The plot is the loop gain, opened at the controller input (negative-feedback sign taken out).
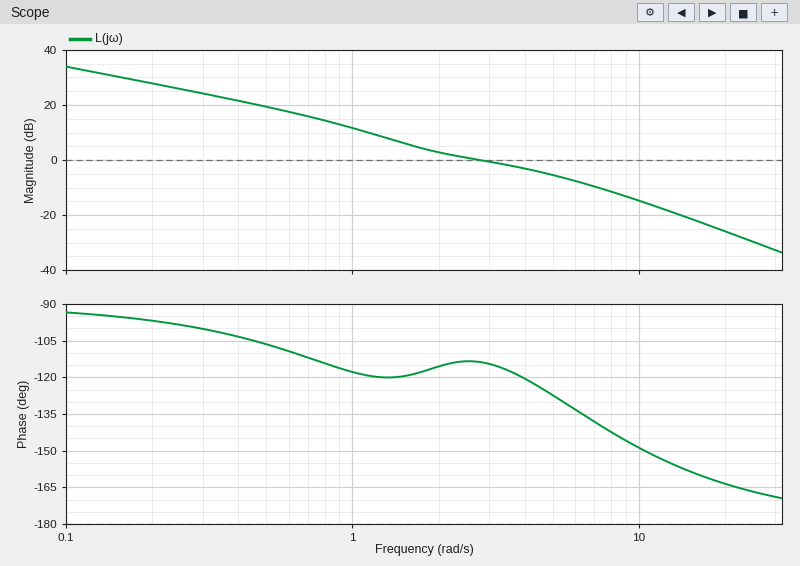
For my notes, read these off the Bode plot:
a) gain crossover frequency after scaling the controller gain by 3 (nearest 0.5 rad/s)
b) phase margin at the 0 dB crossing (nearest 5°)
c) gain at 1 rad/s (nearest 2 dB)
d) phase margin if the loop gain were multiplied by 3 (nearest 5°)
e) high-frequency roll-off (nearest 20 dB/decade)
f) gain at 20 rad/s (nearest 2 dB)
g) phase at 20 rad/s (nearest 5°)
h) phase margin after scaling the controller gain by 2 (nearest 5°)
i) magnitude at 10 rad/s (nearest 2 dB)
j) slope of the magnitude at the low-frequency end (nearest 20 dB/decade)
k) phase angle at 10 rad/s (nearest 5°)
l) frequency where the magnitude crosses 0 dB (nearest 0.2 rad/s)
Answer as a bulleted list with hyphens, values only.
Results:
- 7.0 rad/s
- 65°
- 12 dB
- 40°
- -40 dB/decade
- -26 dB
- -165°
- 50°
- -14 dB
- -20 dB/decade
- -150°
- 2.8 rad/s
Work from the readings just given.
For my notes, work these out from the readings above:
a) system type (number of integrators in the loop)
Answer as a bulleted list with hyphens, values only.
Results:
- 1
